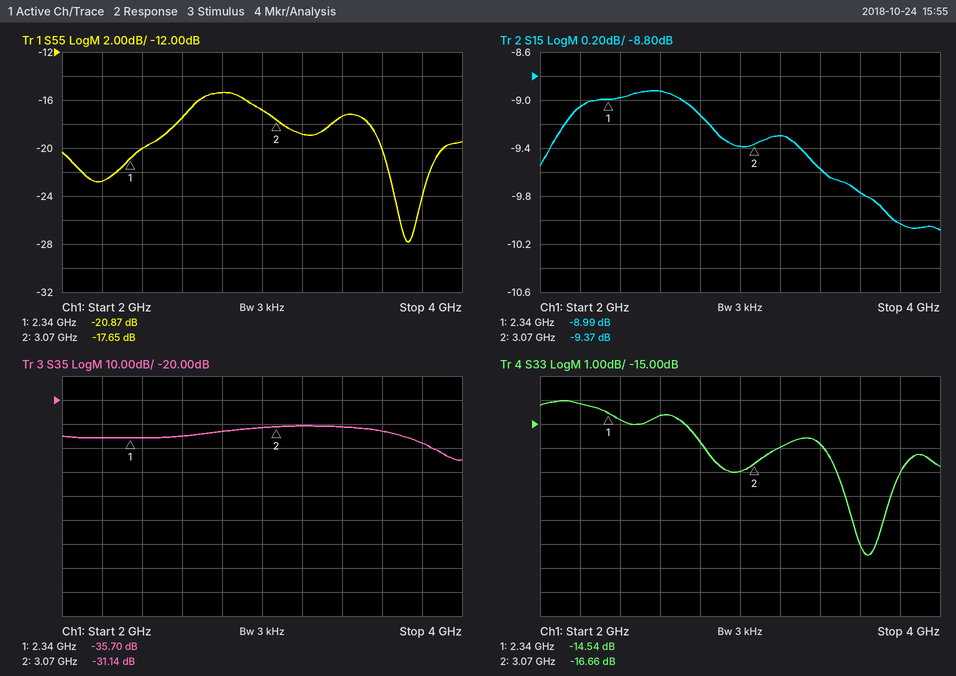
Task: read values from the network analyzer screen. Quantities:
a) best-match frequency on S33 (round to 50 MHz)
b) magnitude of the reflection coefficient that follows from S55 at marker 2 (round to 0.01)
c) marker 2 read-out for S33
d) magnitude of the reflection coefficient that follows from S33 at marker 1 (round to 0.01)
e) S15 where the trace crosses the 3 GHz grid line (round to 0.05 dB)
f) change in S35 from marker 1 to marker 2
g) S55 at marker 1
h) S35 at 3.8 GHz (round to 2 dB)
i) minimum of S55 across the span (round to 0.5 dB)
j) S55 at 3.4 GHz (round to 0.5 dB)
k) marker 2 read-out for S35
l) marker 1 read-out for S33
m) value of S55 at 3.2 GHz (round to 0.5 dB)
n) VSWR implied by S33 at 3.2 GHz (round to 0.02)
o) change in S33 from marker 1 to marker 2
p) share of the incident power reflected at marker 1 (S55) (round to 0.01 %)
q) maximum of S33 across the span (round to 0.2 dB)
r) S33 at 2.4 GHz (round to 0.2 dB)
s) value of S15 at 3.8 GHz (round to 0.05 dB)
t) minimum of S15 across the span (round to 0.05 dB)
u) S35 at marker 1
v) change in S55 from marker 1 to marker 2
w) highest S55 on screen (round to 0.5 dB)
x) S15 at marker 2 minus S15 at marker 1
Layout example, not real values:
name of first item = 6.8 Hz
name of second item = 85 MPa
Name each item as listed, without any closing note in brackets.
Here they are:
best-match frequency on S33 = 3.65 GHz
magnitude of the reflection coefficient that follows from S55 at marker 2 = 0.13
marker 2 read-out for S33 = -16.66 dB
magnitude of the reflection coefficient that follows from S33 at marker 1 = 0.19
S15 where the trace crosses the 3 GHz grid line = -9.40 dB
change in S35 from marker 1 to marker 2 = 4.56 dB
S55 at marker 1 = -20.87 dB
S35 at 3.8 GHz = -38 dB
minimum of S55 across the span = -28.0 dB
S55 at 3.4 GHz = -17.5 dB
marker 2 read-out for S35 = -31.14 dB
marker 1 read-out for S33 = -14.54 dB
value of S55 at 3.2 GHz = -19.0 dB
VSWR implied by S33 at 3.2 GHz = 1.38
change in S33 from marker 1 to marker 2 = -2.12 dB
share of the incident power reflected at marker 1 (S55) = 0.82 %
maximum of S33 across the span = -14.0 dB
S33 at 2.4 GHz = -14.8 dB
value of S15 at 3.8 GHz = -10.05 dB
minimum of S15 across the span = -10.10 dB
S35 at marker 1 = -35.70 dB
change in S55 from marker 1 to marker 2 = 3.22 dB
highest S55 on screen = -15.5 dB
S15 at marker 2 minus S15 at marker 1 = -0.38 dB
